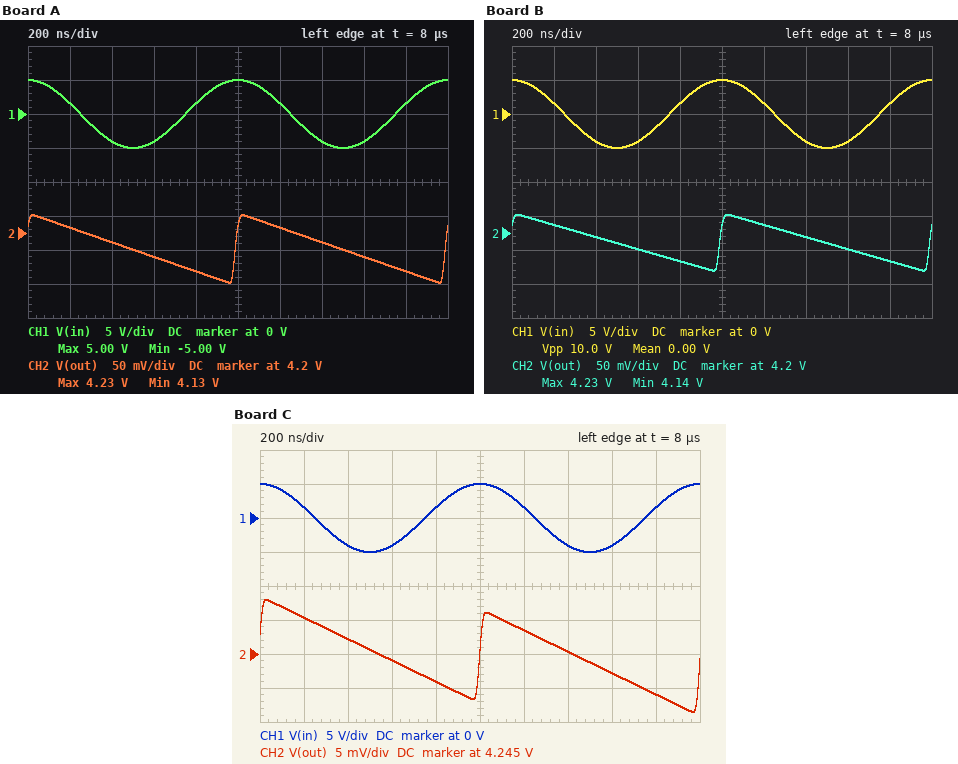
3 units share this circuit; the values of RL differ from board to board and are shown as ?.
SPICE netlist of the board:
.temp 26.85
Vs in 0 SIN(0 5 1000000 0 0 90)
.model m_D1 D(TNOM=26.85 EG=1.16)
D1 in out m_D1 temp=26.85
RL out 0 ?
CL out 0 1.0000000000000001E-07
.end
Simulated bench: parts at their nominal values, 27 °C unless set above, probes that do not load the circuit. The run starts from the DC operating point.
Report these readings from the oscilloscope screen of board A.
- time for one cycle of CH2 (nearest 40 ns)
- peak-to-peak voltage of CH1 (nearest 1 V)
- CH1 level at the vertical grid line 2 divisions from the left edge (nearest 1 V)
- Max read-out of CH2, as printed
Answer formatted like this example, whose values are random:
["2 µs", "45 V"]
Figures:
["1.00 µs", "10 V", "-4 V", "4.23 V"]
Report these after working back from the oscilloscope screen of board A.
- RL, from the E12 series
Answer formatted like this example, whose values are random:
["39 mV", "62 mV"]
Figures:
["390 Ω"]
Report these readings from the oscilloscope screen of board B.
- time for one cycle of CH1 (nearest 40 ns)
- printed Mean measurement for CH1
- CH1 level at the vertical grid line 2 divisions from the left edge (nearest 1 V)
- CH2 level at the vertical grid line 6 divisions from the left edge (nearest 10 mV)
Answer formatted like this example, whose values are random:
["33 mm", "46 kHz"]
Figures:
["1.00 µs", "0.00 V", "-4 V", "4.21 V"]
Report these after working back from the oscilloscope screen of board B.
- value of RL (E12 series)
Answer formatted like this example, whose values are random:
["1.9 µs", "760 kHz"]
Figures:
["470 Ω"]
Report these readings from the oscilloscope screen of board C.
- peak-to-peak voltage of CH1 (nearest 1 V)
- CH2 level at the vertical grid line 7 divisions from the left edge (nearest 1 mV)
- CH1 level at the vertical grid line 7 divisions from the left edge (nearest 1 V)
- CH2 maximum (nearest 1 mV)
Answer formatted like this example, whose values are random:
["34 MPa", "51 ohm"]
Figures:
["10 V", "4.245 V", "-4 V", "4.253 V"]
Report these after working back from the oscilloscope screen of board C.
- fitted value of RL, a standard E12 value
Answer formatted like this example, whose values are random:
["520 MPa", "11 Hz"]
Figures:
["2.7 kΩ"]
